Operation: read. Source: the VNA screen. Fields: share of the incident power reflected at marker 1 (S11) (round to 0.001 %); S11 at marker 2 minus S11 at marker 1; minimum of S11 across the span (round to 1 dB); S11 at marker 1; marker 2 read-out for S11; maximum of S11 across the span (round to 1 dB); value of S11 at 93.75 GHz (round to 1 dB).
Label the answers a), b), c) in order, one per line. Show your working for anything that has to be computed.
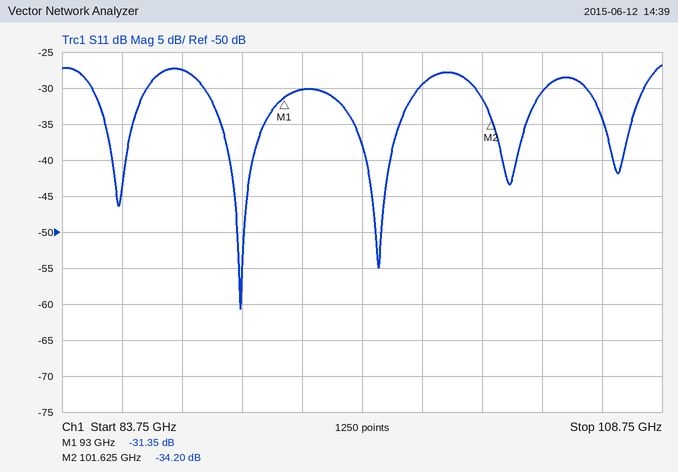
a) 10^(-31.35/10) ≈ 0.073 %
b) -34.2 − (-31.35) = -2.85 dB
c) -61 dB
d) -31.35 dB
e) -34.20 dB
f) -27 dB
g) -30 dB
